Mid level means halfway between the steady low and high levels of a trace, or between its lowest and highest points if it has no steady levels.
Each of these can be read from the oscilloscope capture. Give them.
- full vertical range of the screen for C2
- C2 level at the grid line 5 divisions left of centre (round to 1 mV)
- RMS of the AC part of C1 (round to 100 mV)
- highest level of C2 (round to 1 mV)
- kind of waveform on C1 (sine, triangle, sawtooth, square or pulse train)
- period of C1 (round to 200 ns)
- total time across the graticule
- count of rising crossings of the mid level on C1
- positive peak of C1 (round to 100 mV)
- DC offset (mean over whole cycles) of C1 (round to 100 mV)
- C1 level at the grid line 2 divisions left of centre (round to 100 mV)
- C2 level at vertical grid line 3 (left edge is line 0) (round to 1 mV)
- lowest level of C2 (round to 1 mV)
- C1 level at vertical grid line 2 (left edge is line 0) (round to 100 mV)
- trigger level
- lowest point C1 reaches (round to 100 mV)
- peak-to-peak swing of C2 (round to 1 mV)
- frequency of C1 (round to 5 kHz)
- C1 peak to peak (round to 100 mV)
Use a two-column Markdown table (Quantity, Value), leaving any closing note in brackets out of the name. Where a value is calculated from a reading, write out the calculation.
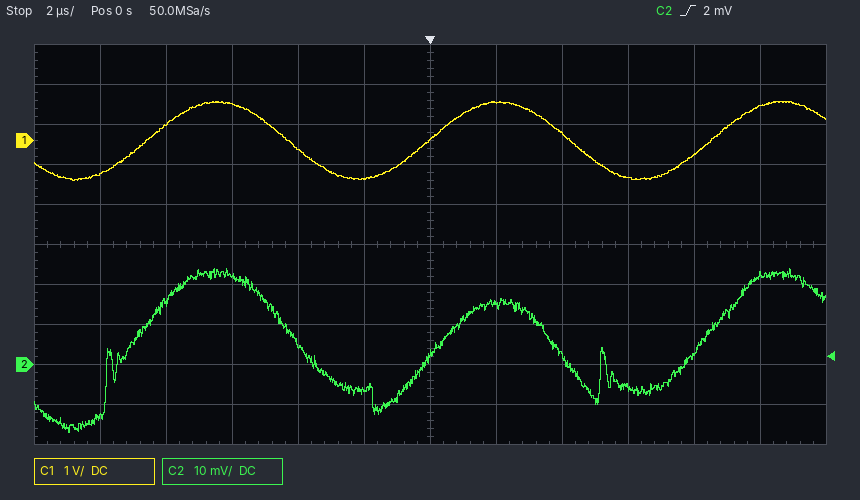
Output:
| Quantity | Value |
|---|---|
| full vertical range of the screen for C2 | 100 mV |
| C2 level at the grid line 5 divisions left of centre | -13 mV |
| RMS of the AC part of C1 | 2.0 V / (2√2) ≈ 707 mV, so 700 mV to the nearest 100 mV |
| highest level of C2 | 24 mV |
| kind of waveform on C1 | sine |
| period of C1 | 8.6 µs |
| total time across the graticule | 24 µs |
| count of rising crossings of the mid level on C1 | 3 |
| positive peak of C1 | 1.0 V |
| DC offset (mean over whole cycles) of C1 | (1.0 V + (-1.0 V)) / 2 ≈ 0.0 V |
| C1 level at the grid line 2 divisions left of centre | -200 mV |
| C2 level at vertical grid line 3 (left edge is line 0) | 22 mV |
| lowest level of C2 | -17 mV |
| C1 level at vertical grid line 2 (left edge is line 0) | 400 mV |
| trigger level | 2 mV |
| lowest point C1 reaches | -1.0 V |
| peak-to-peak swing of C2 | 24 mV − (-17 mV) = 41 mV |
| frequency of C1 | 1 / 8.6 µs ≈ 116 kHz, so 115 kHz to the nearest 5 kHz |
| C1 peak to peak | 1.0 V − (-1.0 V) = 2.0 V |
